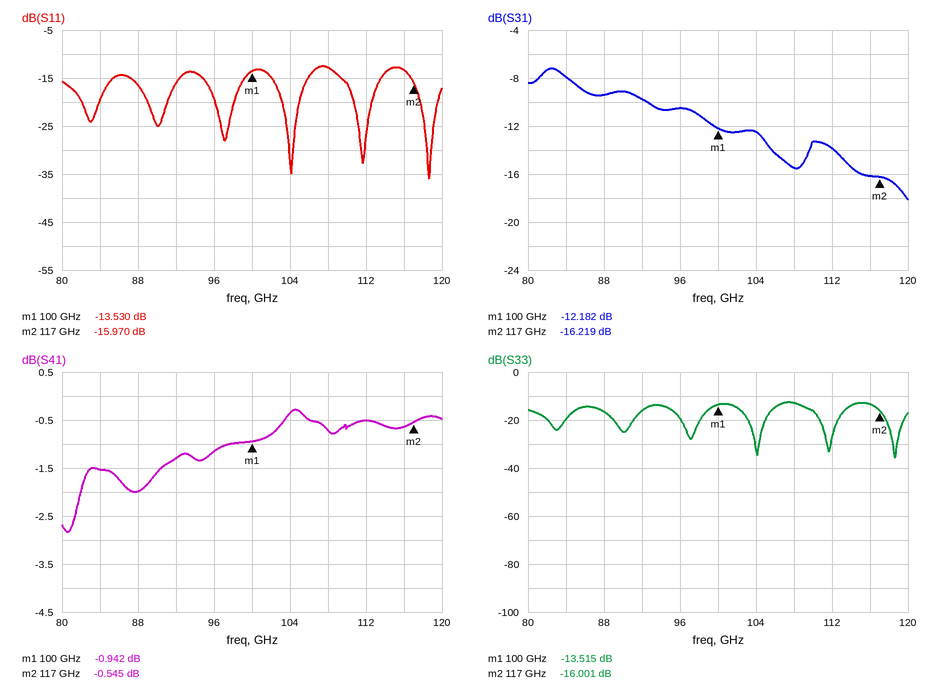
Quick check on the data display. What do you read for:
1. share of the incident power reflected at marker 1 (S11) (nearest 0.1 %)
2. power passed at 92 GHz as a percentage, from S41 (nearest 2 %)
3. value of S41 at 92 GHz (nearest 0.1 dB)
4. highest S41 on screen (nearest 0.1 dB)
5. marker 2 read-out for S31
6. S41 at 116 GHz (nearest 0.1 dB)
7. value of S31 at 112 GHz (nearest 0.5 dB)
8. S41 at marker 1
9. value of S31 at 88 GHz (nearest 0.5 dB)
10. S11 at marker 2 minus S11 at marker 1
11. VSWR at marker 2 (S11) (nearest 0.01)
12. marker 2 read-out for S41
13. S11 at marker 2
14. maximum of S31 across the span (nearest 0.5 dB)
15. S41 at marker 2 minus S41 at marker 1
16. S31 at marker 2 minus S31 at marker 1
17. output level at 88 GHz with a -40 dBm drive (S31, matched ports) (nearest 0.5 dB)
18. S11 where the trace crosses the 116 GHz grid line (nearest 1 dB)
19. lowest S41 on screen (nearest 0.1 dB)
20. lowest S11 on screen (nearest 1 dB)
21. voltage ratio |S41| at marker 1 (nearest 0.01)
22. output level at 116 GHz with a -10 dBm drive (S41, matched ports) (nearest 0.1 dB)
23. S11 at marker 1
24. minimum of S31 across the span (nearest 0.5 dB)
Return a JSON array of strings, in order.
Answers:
["4.4 %", "74 %", "-1.3 dB", "-0.3 dB", "-16.219 dB", "-0.6 dB", "-14.0 dB", "-0.942 dB", "-9.5 dB", "-2.440 dB", "1.38", "-0.545 dB", "-15.970 dB", "-7.0 dB", "0.397 dB", "-4.037 dB", "-49.5 dBm", "-13 dB", "-2.8 dB", "-36 dB", "0.90", "-10.6 dBm", "-13.530 dB", "-18.0 dB"]
